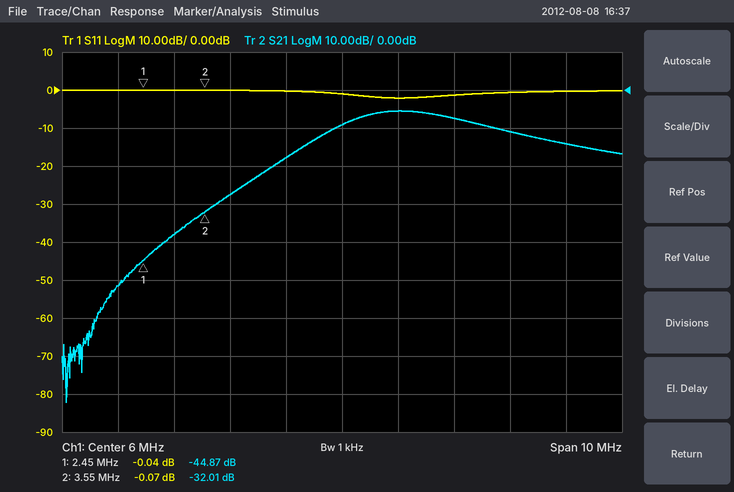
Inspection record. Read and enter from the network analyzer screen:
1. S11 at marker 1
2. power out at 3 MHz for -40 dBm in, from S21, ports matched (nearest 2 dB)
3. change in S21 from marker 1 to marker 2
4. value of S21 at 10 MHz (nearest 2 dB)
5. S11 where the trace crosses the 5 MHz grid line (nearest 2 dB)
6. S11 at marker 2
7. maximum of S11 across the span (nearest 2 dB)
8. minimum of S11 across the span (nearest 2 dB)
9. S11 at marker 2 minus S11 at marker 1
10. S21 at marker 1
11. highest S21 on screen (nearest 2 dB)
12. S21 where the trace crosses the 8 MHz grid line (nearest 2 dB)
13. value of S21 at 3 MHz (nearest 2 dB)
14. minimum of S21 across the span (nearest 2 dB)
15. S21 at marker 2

-0.04 dB
-78 dBm
12.86 dB
-14 dB
0 dB
-0.07 dB
0 dB
-2 dB
-0.03 dB
-44.87 dB
-6 dB
-8 dB
-38 dB
-82 dB
-32.01 dB
